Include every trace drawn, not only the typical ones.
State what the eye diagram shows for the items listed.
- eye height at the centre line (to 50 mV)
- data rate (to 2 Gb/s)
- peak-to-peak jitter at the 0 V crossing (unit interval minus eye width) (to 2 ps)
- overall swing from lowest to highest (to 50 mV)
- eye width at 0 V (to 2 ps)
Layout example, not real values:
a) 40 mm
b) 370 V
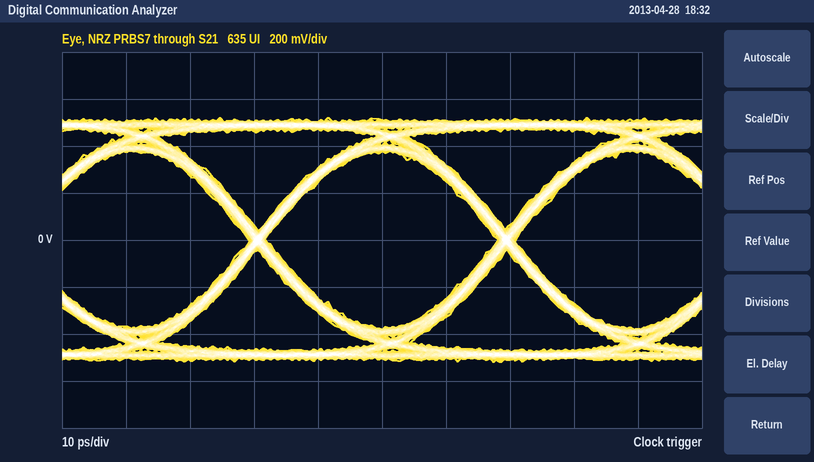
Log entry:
a) 750 mV
b) 26 Gb/s
c) 2 ps
d) 1.05 V
e) 36 ps
